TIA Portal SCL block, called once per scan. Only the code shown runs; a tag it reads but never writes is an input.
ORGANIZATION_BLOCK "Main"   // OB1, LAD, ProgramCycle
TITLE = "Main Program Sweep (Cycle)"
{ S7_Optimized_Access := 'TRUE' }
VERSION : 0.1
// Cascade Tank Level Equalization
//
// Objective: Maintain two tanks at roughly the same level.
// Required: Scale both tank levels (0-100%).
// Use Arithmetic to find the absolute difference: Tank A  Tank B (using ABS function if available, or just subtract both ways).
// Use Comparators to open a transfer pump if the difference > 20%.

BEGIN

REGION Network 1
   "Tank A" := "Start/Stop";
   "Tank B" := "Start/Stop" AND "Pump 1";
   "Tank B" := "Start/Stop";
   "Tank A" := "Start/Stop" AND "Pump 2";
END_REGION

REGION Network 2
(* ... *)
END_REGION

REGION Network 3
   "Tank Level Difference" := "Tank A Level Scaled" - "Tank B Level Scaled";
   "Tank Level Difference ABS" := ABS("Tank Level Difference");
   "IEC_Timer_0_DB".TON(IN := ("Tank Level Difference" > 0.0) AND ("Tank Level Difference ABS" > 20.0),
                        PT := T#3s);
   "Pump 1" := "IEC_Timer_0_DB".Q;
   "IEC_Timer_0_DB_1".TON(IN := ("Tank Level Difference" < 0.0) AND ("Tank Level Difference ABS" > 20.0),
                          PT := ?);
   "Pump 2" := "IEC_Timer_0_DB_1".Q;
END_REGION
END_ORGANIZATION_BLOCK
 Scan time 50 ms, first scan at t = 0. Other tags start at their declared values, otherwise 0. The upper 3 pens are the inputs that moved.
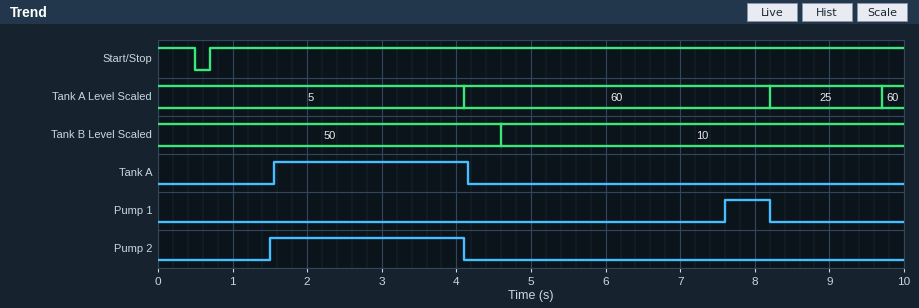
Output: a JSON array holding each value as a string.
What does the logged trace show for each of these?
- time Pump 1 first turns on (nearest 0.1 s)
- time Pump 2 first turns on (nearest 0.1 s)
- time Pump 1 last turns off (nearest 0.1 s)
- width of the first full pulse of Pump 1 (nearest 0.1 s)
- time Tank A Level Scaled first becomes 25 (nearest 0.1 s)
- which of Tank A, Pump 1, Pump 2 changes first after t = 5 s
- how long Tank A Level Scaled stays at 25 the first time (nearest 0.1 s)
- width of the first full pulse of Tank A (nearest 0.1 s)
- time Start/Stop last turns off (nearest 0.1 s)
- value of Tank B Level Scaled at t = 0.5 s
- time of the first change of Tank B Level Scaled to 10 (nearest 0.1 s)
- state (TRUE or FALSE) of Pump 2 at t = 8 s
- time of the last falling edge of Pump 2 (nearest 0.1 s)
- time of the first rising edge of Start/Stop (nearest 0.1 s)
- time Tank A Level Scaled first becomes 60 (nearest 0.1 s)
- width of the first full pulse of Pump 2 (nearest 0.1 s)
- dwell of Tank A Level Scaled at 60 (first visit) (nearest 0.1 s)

["7.6 s", "1.5 s", "8.2 s", "0.6 s", "8.2 s", "Pump 1", "1.5 s", "2.6 s", "0.5 s", "50", "4.6 s", "FALSE", "4.1 s", "0.7 s", "4.1 s", "2.6 s", "4.1 s"]
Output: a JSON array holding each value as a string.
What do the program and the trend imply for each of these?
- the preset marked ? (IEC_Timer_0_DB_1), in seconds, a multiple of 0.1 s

["1.5 s"]
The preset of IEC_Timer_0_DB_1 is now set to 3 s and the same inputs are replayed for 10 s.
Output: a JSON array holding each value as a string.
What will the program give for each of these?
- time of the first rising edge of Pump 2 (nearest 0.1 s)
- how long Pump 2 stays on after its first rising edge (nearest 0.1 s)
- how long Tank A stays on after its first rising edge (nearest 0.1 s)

["3.0 s", "1.1 s", "1.1 s"]
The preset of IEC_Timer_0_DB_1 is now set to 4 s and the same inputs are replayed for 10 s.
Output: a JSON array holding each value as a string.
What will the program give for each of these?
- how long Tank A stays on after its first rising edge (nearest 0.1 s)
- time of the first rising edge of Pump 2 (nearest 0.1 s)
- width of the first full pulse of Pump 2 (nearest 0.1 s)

["0.1 s", "4.0 s", "0.1 s"]
